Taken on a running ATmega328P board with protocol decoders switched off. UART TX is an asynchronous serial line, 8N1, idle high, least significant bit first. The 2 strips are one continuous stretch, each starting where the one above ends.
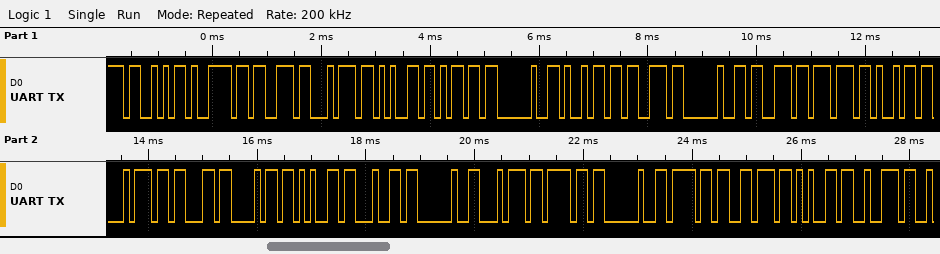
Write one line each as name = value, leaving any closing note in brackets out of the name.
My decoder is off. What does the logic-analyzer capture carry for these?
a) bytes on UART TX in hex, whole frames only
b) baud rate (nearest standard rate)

bytes on UART TX in hex, whole frames only = 53 79 73 74 65 6D 20 69 73 20 73 77 69 74 63 68 65 64 20 74 6F 20 6F 76 65 72
baud rate = 9600 baud
